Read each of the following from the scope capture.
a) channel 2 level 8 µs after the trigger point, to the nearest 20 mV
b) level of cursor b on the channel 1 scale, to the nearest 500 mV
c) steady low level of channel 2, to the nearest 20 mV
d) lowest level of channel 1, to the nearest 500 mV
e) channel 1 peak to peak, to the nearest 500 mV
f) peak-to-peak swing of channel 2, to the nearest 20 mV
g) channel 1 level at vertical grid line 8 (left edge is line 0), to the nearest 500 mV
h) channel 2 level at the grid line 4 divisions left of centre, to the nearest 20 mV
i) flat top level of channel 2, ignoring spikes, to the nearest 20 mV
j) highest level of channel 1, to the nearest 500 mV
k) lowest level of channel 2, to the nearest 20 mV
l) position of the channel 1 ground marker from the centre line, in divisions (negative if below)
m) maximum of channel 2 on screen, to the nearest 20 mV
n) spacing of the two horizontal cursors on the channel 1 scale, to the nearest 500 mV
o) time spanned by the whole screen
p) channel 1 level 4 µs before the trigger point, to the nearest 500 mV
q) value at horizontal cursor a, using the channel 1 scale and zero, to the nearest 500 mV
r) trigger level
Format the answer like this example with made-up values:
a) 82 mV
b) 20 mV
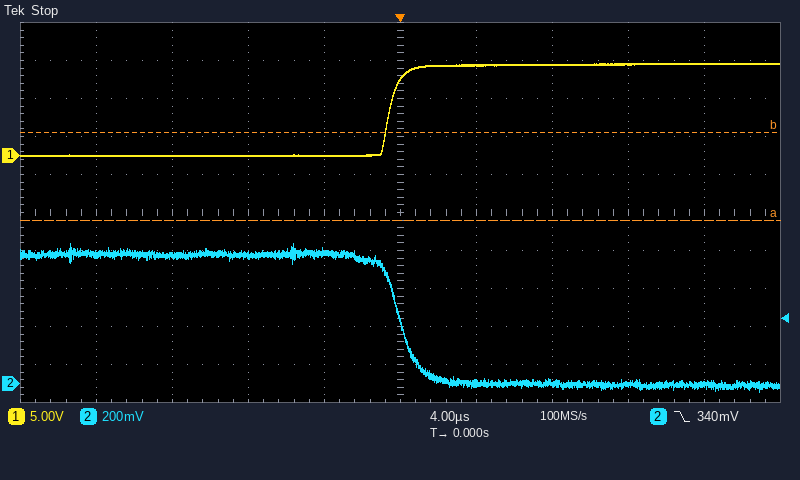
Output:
a) 0 mV
b) 3.0 V
c) 0 mV
d) 0.0 V
e) 12.0 V
f) 780 mV
g) 12.0 V
h) 680 mV
i) 680 mV
j) 12.0 V
k) -40 mV
l) +1.5 div
m) 740 mV
n) 11.5 V
o) 40 µs
p) 0.0 V
q) -8.5 V
r) 340 mV
